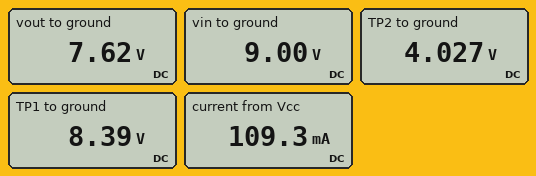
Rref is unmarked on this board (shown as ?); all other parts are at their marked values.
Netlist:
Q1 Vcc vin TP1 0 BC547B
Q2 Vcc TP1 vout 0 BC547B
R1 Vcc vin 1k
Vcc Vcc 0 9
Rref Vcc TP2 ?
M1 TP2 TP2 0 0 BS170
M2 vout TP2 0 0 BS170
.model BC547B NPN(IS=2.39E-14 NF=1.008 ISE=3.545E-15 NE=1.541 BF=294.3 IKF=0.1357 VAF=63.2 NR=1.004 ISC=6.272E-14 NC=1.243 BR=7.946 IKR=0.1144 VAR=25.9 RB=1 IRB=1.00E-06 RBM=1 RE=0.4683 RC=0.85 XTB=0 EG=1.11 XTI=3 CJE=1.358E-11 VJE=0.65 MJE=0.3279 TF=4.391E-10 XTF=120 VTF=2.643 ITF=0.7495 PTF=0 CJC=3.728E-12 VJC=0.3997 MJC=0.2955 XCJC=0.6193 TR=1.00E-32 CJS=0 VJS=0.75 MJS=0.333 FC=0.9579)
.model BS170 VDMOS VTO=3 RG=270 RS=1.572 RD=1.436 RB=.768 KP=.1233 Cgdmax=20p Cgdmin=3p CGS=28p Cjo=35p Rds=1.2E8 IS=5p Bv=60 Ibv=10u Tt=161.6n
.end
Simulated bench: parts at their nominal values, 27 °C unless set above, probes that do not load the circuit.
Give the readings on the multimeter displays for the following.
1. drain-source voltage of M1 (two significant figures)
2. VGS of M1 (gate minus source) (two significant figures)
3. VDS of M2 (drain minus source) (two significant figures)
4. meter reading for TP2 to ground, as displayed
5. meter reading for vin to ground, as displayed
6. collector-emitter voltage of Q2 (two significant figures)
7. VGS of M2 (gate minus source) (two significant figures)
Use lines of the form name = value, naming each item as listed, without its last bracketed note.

drain-source voltage of M1 = 4.0 V
VGS of M1 (gate minus source) = 4.0 V
VDS of M2 (drain minus source) = 7.6 V
meter reading for TP2 to ground, as displayed = 4.027 V
meter reading for vin to ground, as displayed = 9.00 V
collector-emitter voltage of Q2 = 1.4 V
VGS of M2 (gate minus source) = 4.0 V
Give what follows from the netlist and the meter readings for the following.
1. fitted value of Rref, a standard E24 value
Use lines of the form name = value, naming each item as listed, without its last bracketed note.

fitted value of Rref, a standard E24 value = 91 Ω
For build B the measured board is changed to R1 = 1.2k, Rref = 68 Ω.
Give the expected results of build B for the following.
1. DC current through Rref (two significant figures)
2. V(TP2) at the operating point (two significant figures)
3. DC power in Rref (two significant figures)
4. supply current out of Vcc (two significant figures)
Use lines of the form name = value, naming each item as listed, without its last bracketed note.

DC current through Rref = 71 mA
V(TP2) at the operating point = 4.2 V
DC power in Rref = 340 mW
supply current out of Vcc = 140 mA
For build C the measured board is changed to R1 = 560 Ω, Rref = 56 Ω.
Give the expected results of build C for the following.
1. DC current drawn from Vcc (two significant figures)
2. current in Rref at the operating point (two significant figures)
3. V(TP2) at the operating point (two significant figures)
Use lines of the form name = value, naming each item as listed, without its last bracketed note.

DC current drawn from Vcc = 170 mA
current in Rref at the operating point = 84 mA
V(TP2) at the operating point = 4.3 V
